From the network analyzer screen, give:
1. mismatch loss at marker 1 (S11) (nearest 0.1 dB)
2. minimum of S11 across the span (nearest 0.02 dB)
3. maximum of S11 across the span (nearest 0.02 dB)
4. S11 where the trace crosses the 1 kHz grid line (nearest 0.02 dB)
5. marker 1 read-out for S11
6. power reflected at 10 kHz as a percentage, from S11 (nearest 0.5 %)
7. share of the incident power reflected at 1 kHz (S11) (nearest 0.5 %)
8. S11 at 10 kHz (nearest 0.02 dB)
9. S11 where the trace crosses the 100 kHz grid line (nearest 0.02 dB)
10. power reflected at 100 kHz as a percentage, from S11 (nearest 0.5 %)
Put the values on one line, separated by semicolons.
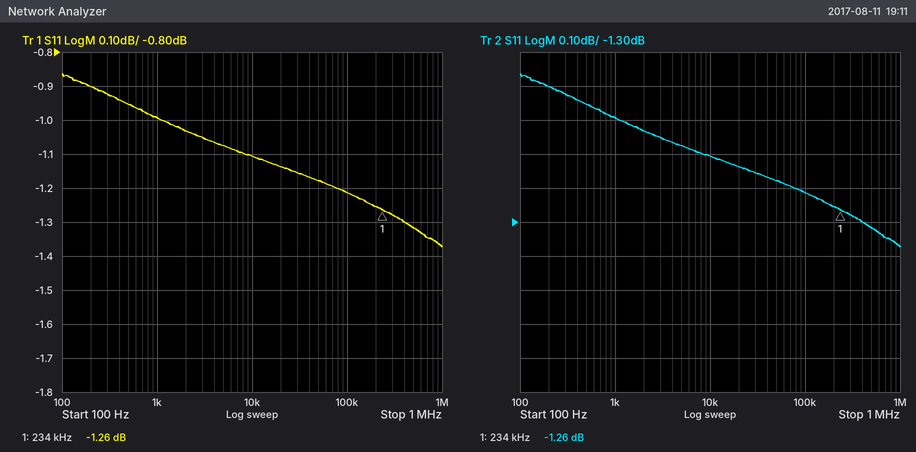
6.0 dB; -1.38 dB; -0.86 dB; -1.00 dB; -1.26 dB; 77.5 %; 79.5 %; -1.10 dB; -1.22 dB; 75.5 %
